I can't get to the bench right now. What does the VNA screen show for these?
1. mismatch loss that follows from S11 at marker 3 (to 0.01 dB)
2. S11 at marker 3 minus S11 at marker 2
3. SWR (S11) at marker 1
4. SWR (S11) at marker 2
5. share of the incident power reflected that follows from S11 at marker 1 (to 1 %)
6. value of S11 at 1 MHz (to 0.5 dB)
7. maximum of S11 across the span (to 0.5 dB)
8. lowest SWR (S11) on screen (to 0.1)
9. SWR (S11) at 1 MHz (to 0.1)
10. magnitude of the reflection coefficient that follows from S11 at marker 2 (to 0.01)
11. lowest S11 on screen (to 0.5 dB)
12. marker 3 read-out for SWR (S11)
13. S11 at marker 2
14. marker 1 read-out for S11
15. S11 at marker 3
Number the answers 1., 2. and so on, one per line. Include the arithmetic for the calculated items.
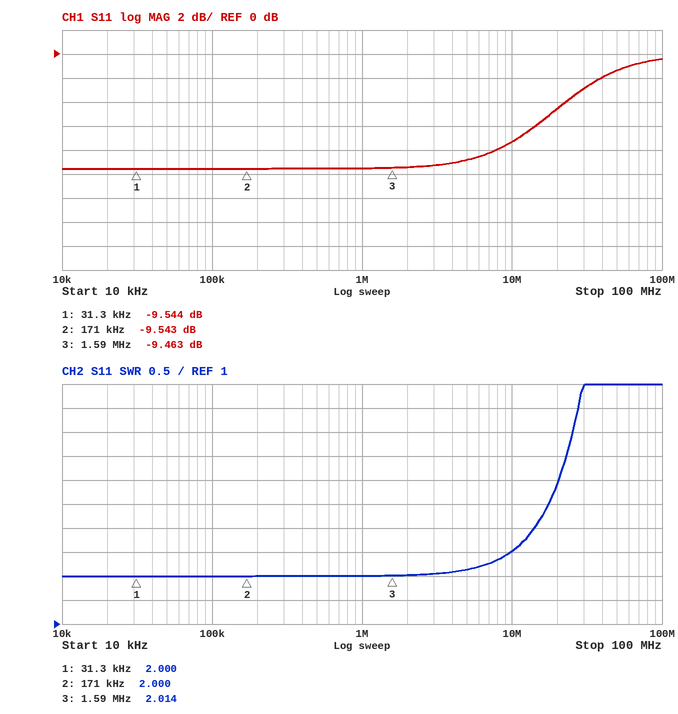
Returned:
1. −10 log10(1 − 10^(-9.463/10)) ≈ 0.52 dB
2. -9.463 − (-9.543) = 0.080 dB
3. 2.000
4. 2.000
5. 10^(-9.544/10) ≈ 11 %
6. -9.5 dB
7. -0.5 dB
8. 2.0
9. 2.0
10. 10^(-9.543/20) ≈ 0.33
11. -9.5 dB
12. 2.014
13. -9.543 dB
14. -9.544 dB
15. -9.463 dB
